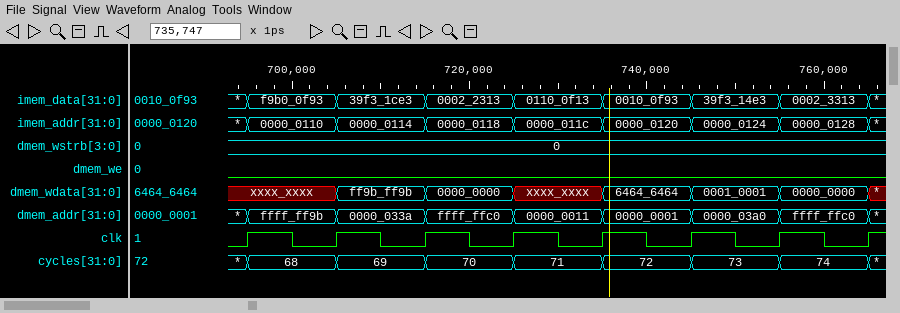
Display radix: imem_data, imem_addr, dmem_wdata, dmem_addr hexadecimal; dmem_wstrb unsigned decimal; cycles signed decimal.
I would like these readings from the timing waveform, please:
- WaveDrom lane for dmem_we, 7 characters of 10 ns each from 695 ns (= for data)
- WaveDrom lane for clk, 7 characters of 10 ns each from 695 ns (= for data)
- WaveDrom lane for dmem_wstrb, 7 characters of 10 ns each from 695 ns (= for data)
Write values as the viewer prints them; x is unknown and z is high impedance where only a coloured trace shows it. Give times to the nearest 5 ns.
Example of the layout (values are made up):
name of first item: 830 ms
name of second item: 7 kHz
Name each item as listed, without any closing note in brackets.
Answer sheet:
WaveDrom lane for dmem_we, 7 characters of 10 ns each from 695 ns: {name: 'dmem_we', wave: '0......'}
WaveDrom lane for clk, 7 characters of 10 ns each from 695 ns: {name: 'clk', wave: 'p......'}
WaveDrom lane for dmem_wstrb, 7 characters of 10 ns each from 695 ns: {name: 'dmem_wstrb', wave: '=......', data: '0'}
